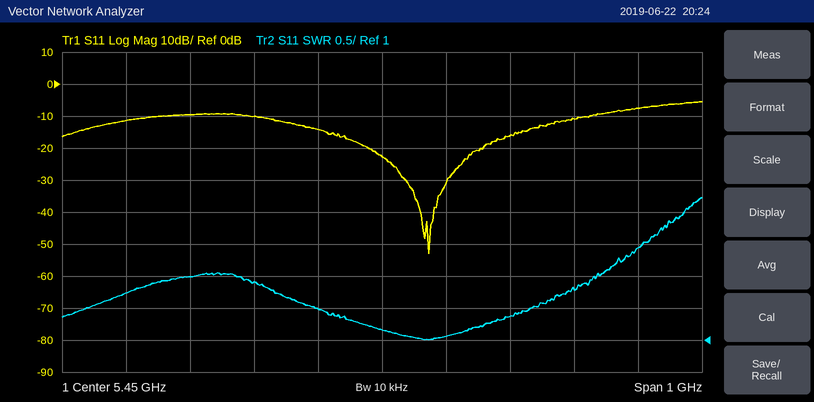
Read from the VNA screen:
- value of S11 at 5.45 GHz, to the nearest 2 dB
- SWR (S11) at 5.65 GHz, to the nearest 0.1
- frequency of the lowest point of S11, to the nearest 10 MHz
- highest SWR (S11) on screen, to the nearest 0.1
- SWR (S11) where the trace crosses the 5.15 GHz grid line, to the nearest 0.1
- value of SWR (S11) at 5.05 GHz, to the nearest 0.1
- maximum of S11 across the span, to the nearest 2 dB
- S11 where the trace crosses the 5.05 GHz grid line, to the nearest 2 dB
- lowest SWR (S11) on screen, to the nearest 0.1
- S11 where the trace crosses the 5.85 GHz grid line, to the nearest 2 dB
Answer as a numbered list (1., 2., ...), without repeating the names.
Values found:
1. -22 dB
2. 1.4
3. 5.52 GHz
4. 3.2
5. 2.0
6. 1.7
7. -6 dB
8. -12 dB
9. 1.0
10. -8 dB
